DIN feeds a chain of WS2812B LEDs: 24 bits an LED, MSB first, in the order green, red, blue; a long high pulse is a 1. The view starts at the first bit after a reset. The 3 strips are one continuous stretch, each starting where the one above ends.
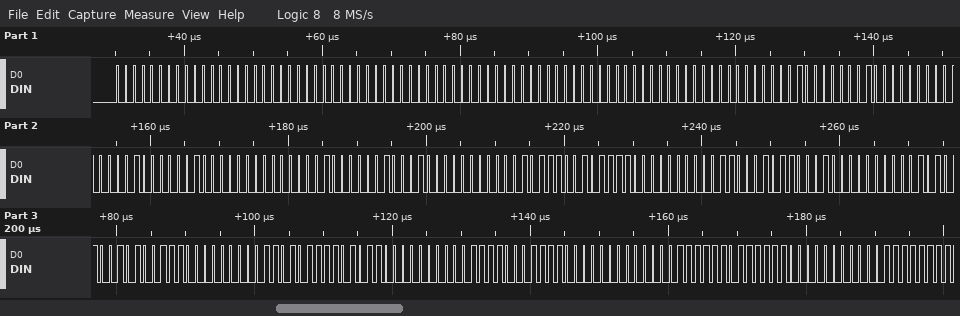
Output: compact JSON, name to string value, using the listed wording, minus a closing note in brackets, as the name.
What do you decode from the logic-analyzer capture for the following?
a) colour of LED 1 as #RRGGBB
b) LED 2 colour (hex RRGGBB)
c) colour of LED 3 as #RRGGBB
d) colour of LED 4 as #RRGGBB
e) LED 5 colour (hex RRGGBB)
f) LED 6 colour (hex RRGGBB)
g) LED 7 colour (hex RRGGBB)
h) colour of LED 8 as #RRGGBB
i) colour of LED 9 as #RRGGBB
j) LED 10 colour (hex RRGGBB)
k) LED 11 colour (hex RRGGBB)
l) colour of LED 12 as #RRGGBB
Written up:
{"colour of LED 1 as #RRGGBB": "#000000", "LED 2 colour": "#000000", "colour of LED 3 as #RRGGBB": "#000000", "colour of LED 4 as #RRGGBB": "#010100", "LED 5 colour": "#040200", "LED 6 colour": "#110800", "LED 7 colour": "#2F1700", "colour of LED 8 as #RRGGBB": "#623100", "colour of LED 9 as #RRGGBB": "#A75400", "LED 10 colour": "#D66B00", "LED 11 colour": "#F07800", "colour of LED 12 as #RRGGBB": "#FC7E00"}
